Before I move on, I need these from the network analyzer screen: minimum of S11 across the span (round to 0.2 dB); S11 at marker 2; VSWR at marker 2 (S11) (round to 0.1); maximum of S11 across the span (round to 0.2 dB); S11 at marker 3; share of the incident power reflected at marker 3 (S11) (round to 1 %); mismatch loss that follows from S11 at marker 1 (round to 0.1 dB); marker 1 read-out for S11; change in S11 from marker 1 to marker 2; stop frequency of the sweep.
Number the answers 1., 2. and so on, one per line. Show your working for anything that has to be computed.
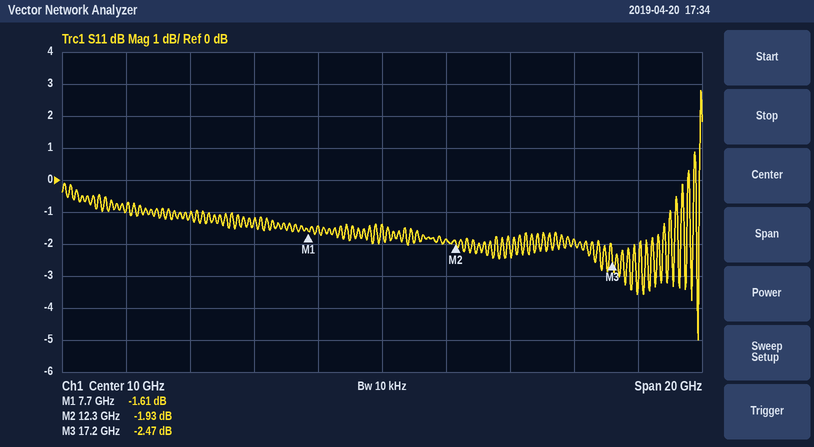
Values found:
1. -5.0 dB
2. -1.93 dB
3. (1 + 0.8008)/(1 − 0.8008) ≈ 9.0
4. 2.8 dB
5. -2.47 dB
6. 10^(-2.47/10) ≈ 57 %
7. −10 log10(1 − 10^(-1.61/10)) ≈ 5.1 dB
8. -1.61 dB
9. -1.93 − (-1.61) = -0.32 dB
10. 20 GHz
